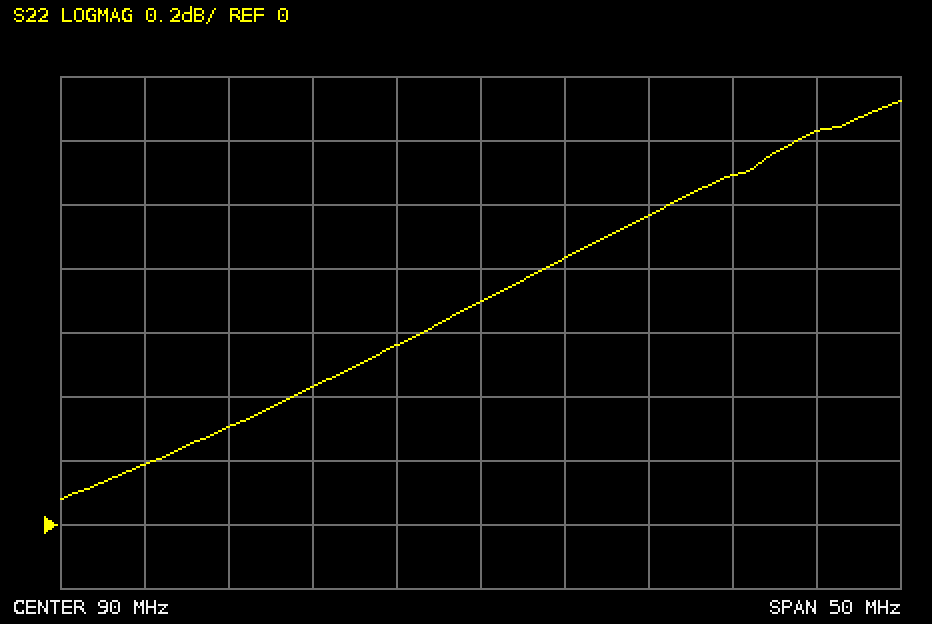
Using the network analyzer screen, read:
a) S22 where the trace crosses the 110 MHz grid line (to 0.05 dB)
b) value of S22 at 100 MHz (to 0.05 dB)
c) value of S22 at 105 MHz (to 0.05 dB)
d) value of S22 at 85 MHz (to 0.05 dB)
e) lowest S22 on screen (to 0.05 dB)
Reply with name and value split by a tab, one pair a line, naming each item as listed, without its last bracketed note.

S22 where the trace crosses the 110 MHz grid line	1.25 dB
value of S22 at 100 MHz	0.95 dB
value of S22 at 105 MHz	1.10 dB
value of S22 at 85 MHz	0.55 dB
lowest S22 on screen	0.10 dB
